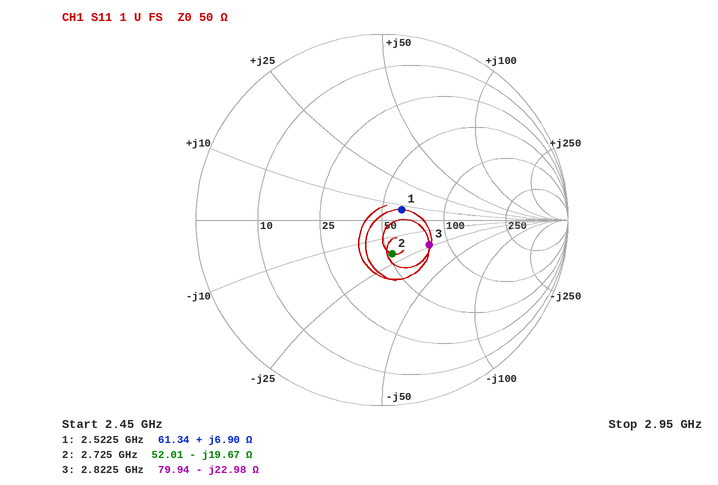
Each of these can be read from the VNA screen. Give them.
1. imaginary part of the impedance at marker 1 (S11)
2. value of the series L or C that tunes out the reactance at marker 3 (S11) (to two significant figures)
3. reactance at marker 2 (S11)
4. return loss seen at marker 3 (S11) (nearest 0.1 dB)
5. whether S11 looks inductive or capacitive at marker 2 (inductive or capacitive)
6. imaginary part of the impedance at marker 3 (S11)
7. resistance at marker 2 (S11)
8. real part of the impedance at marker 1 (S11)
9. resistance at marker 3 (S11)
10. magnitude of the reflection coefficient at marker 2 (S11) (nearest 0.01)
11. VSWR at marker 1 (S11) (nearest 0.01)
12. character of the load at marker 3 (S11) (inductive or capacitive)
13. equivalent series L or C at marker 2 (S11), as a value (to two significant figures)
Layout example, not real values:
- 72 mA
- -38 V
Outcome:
- +6.90 Ω
- 1.3 nH
- -19.67 Ω
- 10.9 dB
- capacitive
- -22.98 Ω
- 52.01 Ω
- 61.34 Ω
- 79.94 Ω
- 0.19
- 1.27
- capacitive
- 3.0 pF
